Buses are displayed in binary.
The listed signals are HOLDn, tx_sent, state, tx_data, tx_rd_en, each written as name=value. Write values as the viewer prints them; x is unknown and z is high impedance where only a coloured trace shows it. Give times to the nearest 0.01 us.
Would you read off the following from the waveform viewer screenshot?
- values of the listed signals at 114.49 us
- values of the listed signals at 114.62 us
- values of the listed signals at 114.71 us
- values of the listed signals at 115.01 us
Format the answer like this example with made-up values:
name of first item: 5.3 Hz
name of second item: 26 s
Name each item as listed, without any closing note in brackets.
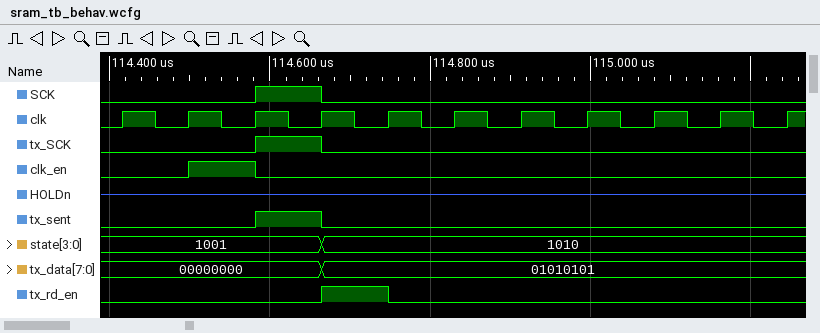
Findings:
values of the listed signals at 114.49 us: HOLDn=z, tx_sent=0, state=1001, tx_data=00000000, tx_rd_en=0
values of the listed signals at 114.62 us: HOLDn=z, tx_sent=1, state=1001, tx_data=00000000, tx_rd_en=0
values of the listed signals at 114.71 us: HOLDn=z, tx_sent=0, state=1010, tx_data=01010101, tx_rd_en=1
values of the listed signals at 115.01 us: HOLDn=z, tx_sent=0, state=1010, tx_data=01010101, tx_rd_en=0
